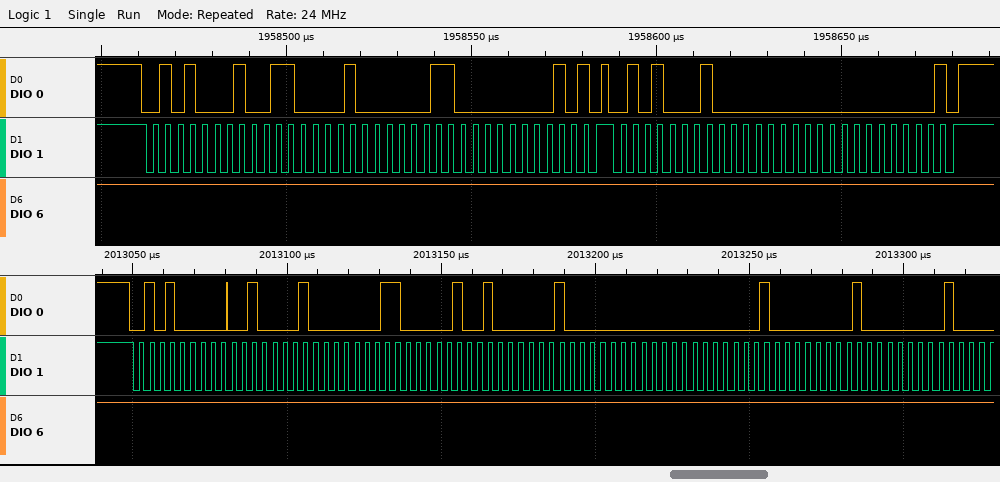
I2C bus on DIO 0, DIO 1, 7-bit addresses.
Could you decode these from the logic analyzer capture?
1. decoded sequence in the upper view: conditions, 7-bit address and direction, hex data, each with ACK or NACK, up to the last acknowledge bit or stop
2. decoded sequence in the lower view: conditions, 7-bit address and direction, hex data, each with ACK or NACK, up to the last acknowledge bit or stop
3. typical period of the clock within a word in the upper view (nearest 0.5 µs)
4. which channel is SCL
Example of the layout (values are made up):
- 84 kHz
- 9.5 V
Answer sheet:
- start, address 28 read ACK, 61 ACK, 06 ACK, 02 NACK, stop, start, address 28 read ACK, 00 ACK, 00 NACK, stop
- start, address 28 write ACK, 21 ACK, 03 ACK, 09 ACK, 04 ACK, 00 ACK, 01 ACK, 01 ACK, 01 ACK
- 3.5 µs
- DIO 1
